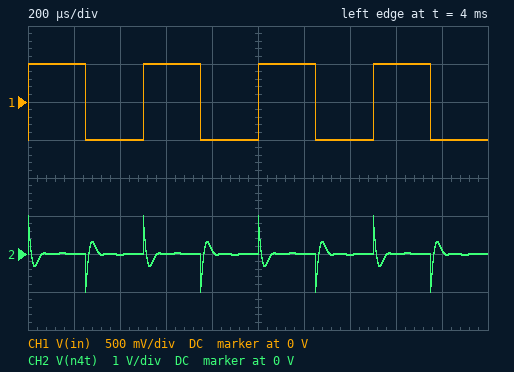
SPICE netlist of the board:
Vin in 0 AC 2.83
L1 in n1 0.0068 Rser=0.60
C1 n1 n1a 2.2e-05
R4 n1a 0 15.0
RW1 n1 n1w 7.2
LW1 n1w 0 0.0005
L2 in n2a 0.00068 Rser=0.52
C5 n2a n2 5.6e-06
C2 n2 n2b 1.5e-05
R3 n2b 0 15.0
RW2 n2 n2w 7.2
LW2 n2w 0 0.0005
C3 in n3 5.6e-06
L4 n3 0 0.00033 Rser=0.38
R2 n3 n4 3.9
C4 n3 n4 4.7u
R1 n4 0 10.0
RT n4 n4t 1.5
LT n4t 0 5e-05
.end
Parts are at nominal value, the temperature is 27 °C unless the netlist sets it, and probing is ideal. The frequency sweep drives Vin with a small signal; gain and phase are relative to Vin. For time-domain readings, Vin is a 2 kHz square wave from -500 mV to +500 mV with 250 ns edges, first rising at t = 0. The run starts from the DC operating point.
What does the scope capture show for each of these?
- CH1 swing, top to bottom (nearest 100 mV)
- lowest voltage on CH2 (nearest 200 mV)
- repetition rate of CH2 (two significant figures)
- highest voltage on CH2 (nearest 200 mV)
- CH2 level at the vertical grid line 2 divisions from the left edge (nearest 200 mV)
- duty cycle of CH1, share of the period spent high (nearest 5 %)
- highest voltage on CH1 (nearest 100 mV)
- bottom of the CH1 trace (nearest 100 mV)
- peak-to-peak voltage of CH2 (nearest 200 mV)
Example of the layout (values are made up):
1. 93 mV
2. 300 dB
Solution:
1. 1.0 V
2. -1.0 V
3. 2.0 kHz
4. 1.0 V
5. 0 V
6. 50 %
7. 500 mV
8. -500 mV
9. 2.0 V
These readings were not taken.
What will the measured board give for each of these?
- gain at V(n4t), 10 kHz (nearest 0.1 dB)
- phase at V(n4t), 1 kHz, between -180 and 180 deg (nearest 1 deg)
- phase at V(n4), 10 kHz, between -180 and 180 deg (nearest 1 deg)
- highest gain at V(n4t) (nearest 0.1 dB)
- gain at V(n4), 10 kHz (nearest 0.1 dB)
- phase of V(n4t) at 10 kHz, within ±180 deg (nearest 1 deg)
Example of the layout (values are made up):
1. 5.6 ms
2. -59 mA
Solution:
1. -3.7 dB
2. -123 deg
3. 89 deg
4. 1.9 dB
5. -2.8 dB
6. 115 deg
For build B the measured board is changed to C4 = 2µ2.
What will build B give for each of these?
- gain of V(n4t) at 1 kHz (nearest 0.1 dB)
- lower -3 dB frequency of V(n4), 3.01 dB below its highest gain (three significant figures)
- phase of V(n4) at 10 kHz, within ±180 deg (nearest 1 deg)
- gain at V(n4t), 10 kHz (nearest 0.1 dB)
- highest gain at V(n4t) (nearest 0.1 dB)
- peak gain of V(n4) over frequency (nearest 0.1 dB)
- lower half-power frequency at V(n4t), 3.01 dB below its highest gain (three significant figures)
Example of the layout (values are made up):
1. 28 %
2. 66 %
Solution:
1. -48.9 dB
2. 13.0 kHz
3. 78 deg
4. -5.3 dB
5. 0.5 dB
6. 0.6 dB
7. 13.7 kHz
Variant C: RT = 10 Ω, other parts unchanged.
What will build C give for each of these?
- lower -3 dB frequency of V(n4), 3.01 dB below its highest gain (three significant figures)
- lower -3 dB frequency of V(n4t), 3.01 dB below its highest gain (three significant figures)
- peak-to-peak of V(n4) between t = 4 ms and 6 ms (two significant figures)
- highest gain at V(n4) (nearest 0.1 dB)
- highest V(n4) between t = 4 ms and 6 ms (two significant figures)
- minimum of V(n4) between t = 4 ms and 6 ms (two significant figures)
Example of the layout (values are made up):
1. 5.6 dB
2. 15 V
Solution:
1. 9.73 kHz
2. 30.7 kHz
3. 1.9 V
4. 0.3 dB
5. 960 mV
6. -960 mV
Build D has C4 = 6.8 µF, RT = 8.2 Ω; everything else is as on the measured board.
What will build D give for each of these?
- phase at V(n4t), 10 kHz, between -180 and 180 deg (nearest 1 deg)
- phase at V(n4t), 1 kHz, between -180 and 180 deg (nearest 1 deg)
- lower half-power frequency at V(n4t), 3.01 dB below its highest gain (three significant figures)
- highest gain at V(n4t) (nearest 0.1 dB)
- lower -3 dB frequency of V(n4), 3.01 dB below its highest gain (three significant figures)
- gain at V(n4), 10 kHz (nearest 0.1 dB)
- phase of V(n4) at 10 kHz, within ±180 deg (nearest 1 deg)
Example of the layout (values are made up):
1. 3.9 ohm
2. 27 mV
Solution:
1. 116 deg
2. -113 deg
3. 24.0 kHz
4. 0 dB
5. 8.96 kHz
6. -2.1 dB
7. 47 deg
